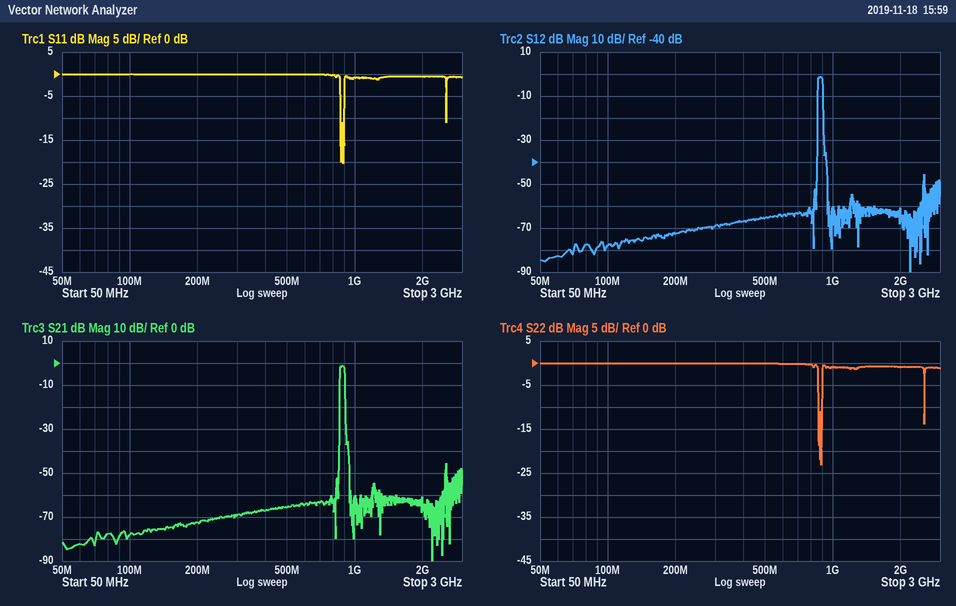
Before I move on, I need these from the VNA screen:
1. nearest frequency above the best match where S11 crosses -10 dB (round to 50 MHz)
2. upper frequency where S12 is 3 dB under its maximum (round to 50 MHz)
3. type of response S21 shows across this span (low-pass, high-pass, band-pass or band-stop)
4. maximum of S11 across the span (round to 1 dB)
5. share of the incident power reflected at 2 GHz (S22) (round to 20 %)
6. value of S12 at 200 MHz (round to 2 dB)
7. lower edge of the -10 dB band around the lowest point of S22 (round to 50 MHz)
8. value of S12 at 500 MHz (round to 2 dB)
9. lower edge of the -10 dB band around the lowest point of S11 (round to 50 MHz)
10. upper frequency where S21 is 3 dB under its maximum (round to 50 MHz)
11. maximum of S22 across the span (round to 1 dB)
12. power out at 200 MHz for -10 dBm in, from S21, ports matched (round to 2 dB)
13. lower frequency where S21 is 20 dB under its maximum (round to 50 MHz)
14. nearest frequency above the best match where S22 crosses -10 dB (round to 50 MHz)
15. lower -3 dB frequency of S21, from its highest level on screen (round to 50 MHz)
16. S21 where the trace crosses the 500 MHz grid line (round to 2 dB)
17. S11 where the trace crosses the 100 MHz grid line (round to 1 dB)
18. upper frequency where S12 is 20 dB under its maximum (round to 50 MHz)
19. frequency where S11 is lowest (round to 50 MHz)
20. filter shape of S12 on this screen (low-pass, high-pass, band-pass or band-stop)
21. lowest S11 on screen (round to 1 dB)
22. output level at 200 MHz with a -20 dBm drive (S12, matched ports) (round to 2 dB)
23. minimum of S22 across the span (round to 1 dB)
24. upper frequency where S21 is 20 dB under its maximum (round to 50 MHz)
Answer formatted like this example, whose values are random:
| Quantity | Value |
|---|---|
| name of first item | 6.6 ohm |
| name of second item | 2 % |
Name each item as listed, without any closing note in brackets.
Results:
| Quantity | Value |
|---|---|
| nearest frequency above the best match where S11 crosses -10 dB | 900 MHz |
| upper frequency where S12 is 3 dB under its maximum | 900 MHz |
| type of response S21 shows across this span | band-pass |
| maximum of S11 across the span | 0 dB |
| share of the incident power reflected at 2 GHz (S22) | 80 % |
| value of S12 at 200 MHz | -72 dB |
| lower edge of the -10 dB band around the lowest point of S22 | 850 MHz |
| value of S12 at 500 MHz | -66 dB |
| lower edge of the -10 dB band around the lowest point of S11 | 850 MHz |
| upper frequency where S21 is 3 dB under its maximum | 900 MHz |
| maximum of S22 across the span | 0 dB |
| power out at 200 MHz for -10 dBm in, from S21, ports matched | -82 dBm |
| lower frequency where S21 is 20 dB under its maximum | 850 MHz |
| nearest frequency above the best match where S22 crosses -10 dB | 900 MHz |
| lower -3 dB frequency of S21, from its highest level on screen | 850 MHz |
| S21 where the trace crosses the 500 MHz grid line | -66 dB |
| S11 where the trace crosses the 100 MHz grid line | 0 dB |
| upper frequency where S12 is 20 dB under its maximum | 900 MHz |
| frequency where S11 is lowest | 900 MHz |
| filter shape of S12 on this screen | band-pass |
| lowest S11 on screen | -20 dB |
| output level at 200 MHz with a -20 dBm drive (S12, matched ports) | -92 dBm |
| minimum of S22 across the span | -23 dB |
| upper frequency where S21 is 20 dB under its maximum | 900 MHz |
